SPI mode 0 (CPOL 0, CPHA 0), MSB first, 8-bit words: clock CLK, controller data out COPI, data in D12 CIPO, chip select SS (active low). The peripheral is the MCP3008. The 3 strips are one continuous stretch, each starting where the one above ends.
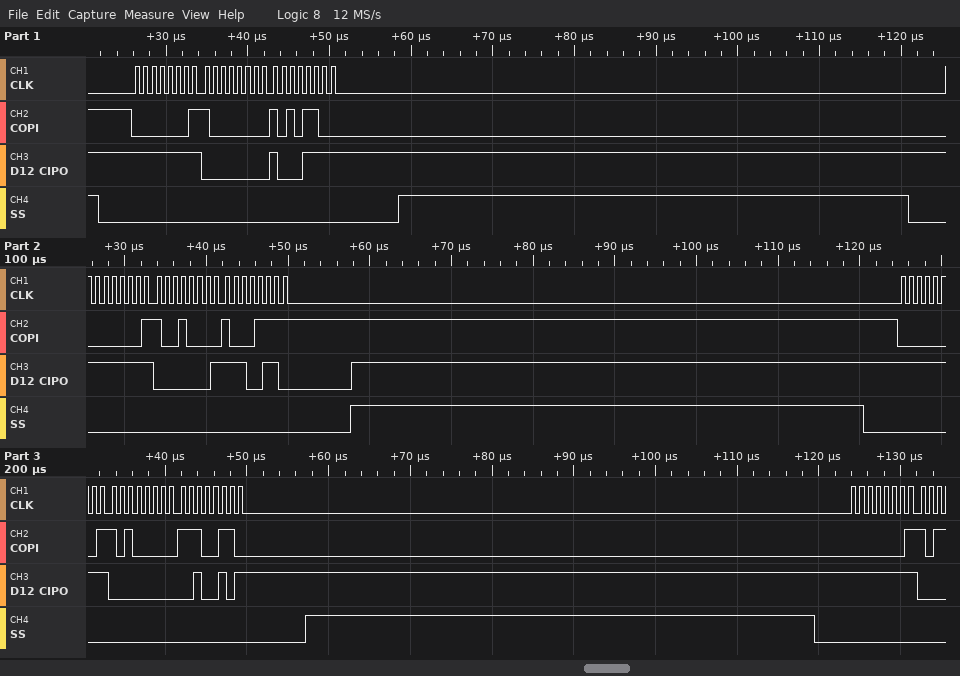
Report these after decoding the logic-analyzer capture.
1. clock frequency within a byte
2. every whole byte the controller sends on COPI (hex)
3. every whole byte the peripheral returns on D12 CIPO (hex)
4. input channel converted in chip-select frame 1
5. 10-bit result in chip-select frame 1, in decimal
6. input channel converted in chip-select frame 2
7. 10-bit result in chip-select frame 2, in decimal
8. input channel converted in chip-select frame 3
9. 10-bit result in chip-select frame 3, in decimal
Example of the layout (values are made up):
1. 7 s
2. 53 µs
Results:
1. 1 MHz
2. 01 80 AC 01 90 8F 01 A0 E6 01
3. FF 00 8F FF 01 E6 FF 00 25 FF
4. 0
5. 143
6. 1
7. 486
8. 2
9. 37
